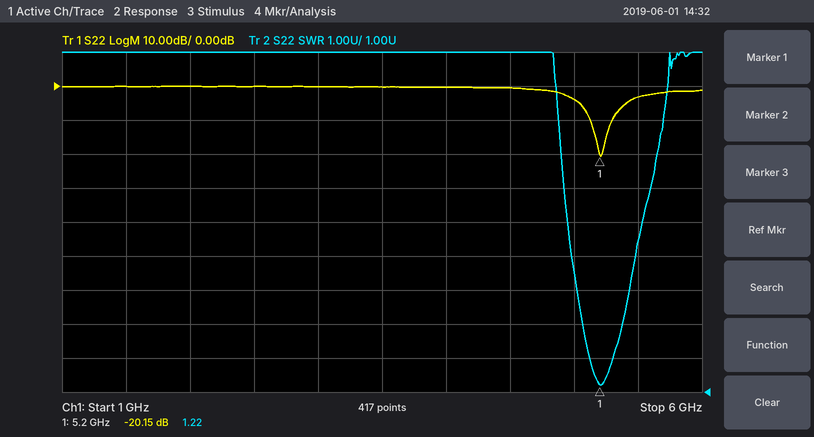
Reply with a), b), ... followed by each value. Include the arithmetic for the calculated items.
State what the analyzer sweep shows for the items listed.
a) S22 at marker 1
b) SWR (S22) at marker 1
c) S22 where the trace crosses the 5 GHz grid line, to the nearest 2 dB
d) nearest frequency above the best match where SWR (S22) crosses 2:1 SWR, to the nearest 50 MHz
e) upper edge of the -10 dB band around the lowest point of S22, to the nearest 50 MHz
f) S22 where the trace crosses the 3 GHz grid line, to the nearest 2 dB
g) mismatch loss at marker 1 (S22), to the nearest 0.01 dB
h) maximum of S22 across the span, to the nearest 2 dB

a) -20.15 dB
b) 1.22
c) -4 dB
d) 5.30 GHz
e) 5.30 GHz
f) 0 dB
g) −10 log10(1 − 10^(-20.15/10)) ≈ 0.04 dB
h) 0 dB
